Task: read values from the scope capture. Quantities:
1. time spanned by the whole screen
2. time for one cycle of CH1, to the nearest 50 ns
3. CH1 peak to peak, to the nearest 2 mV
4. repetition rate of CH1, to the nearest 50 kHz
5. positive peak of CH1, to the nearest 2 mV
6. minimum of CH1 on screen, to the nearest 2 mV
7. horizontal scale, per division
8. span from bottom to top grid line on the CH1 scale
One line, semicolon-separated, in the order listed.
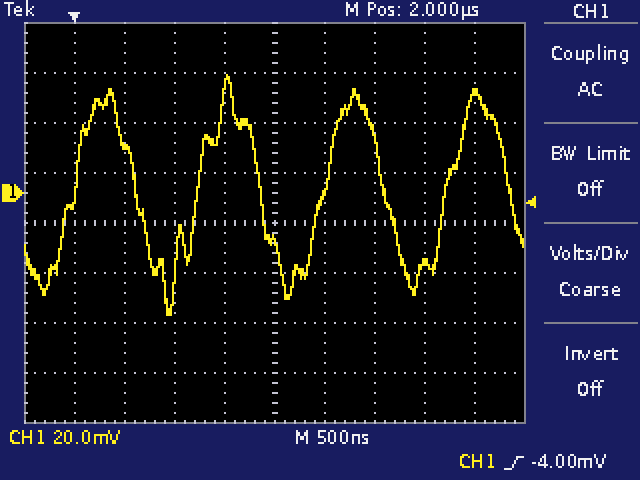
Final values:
5 µs; 1.25 µs; 96 mV; 800 kHz; 48 mV; -48 mV; 500 ns; 160 mV
